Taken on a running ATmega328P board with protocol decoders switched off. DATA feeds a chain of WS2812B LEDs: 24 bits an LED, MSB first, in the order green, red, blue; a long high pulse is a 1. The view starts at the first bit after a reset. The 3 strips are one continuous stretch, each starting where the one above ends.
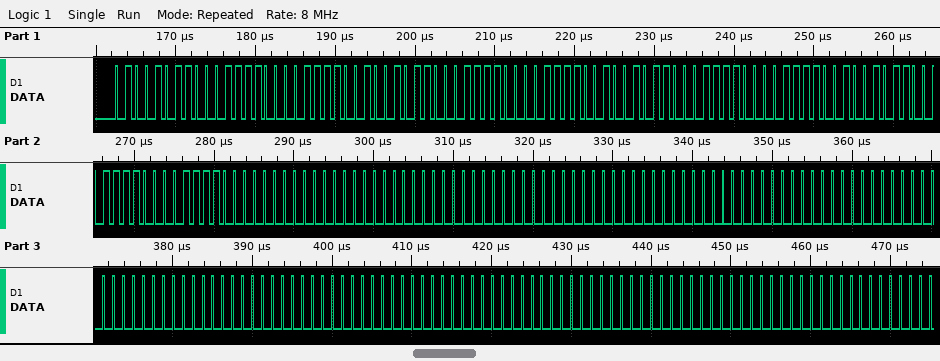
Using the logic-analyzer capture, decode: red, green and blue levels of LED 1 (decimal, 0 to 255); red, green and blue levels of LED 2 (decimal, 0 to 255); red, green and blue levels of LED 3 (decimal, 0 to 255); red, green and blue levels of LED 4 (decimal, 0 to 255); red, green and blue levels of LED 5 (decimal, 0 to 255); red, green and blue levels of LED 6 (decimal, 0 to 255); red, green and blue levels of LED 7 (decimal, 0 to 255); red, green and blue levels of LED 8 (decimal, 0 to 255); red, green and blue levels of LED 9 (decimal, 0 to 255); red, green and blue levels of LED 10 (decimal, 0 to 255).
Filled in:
30, 75, 30
30, 75, 30
30, 75, 30
30, 75, 30
0, 0, 0
0, 0, 0
0, 0, 0
0, 0, 0
0, 0, 0
0, 0, 0
